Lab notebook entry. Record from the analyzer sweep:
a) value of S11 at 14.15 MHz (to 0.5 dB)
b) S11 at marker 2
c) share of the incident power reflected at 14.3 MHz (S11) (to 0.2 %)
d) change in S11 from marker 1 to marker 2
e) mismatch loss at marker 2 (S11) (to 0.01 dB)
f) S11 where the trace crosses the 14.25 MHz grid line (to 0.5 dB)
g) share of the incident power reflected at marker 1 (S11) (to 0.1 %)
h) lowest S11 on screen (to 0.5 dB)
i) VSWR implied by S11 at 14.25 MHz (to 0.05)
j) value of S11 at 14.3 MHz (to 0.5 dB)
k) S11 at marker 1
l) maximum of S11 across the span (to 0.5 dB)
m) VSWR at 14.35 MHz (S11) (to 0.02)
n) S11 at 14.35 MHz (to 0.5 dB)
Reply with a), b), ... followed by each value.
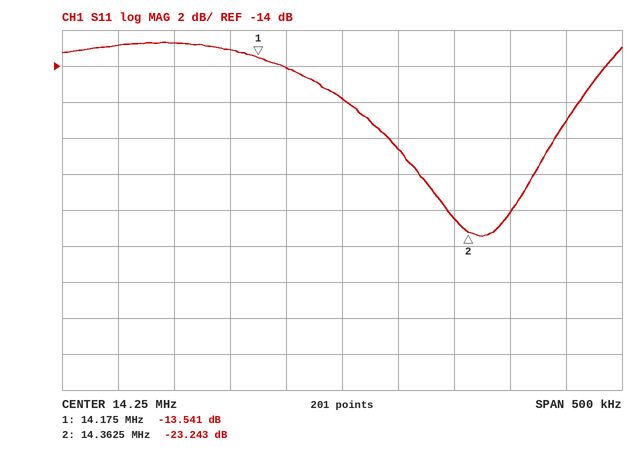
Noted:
a) -13.0 dB
b) -23.243 dB
c) 1.4 %
d) -9.702 dB
e) 0.02 dB
f) -16.0 dB
g) 4.4 %
h) -23.5 dB
i) 1.40
j) -18.5 dB
k) -13.541 dB
l) -12.5 dB
m) 1.16
n) -22.5 dB
